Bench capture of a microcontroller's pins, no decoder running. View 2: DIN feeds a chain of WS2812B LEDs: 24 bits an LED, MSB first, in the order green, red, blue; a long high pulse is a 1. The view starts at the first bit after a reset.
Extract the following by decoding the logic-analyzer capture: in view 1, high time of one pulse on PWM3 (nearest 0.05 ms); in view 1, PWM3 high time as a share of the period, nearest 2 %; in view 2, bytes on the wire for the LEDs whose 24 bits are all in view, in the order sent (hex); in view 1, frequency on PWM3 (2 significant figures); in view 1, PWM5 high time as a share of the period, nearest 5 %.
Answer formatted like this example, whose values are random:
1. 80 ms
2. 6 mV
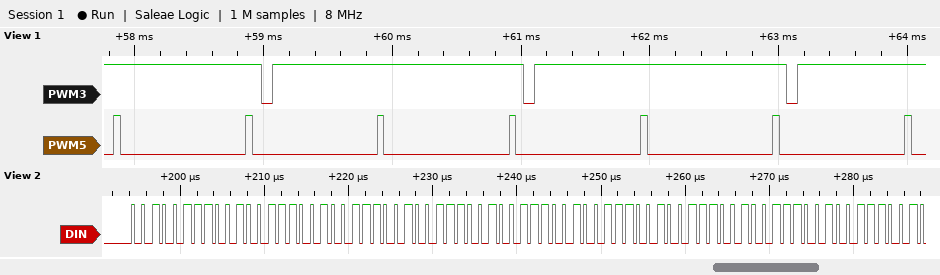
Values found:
1. 1.95 ms
2. 96 %
3. 27 27 27 27 27 27 27 27 27
4. 490 Hz
5. 5 %
